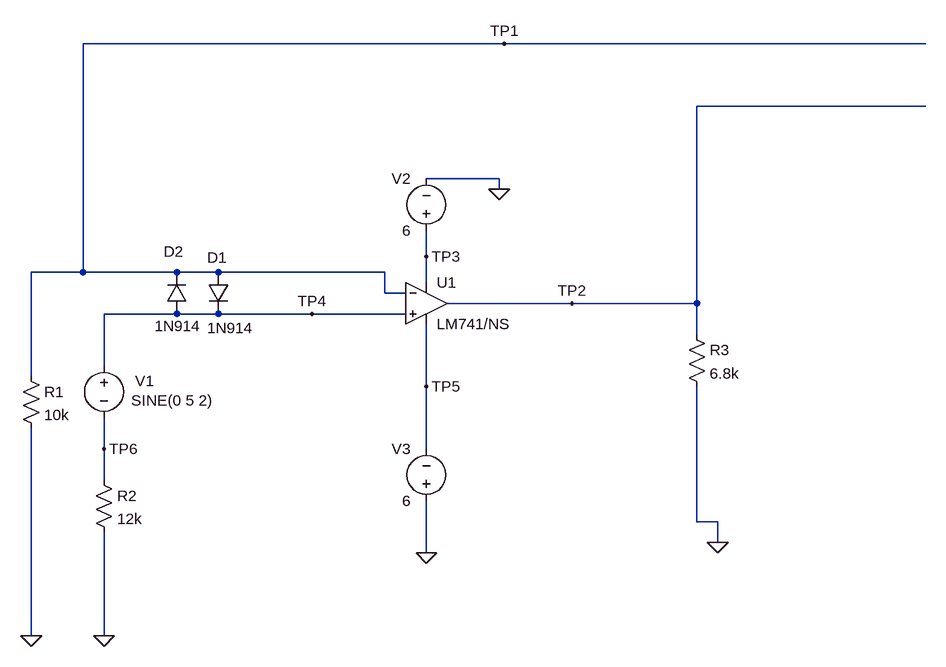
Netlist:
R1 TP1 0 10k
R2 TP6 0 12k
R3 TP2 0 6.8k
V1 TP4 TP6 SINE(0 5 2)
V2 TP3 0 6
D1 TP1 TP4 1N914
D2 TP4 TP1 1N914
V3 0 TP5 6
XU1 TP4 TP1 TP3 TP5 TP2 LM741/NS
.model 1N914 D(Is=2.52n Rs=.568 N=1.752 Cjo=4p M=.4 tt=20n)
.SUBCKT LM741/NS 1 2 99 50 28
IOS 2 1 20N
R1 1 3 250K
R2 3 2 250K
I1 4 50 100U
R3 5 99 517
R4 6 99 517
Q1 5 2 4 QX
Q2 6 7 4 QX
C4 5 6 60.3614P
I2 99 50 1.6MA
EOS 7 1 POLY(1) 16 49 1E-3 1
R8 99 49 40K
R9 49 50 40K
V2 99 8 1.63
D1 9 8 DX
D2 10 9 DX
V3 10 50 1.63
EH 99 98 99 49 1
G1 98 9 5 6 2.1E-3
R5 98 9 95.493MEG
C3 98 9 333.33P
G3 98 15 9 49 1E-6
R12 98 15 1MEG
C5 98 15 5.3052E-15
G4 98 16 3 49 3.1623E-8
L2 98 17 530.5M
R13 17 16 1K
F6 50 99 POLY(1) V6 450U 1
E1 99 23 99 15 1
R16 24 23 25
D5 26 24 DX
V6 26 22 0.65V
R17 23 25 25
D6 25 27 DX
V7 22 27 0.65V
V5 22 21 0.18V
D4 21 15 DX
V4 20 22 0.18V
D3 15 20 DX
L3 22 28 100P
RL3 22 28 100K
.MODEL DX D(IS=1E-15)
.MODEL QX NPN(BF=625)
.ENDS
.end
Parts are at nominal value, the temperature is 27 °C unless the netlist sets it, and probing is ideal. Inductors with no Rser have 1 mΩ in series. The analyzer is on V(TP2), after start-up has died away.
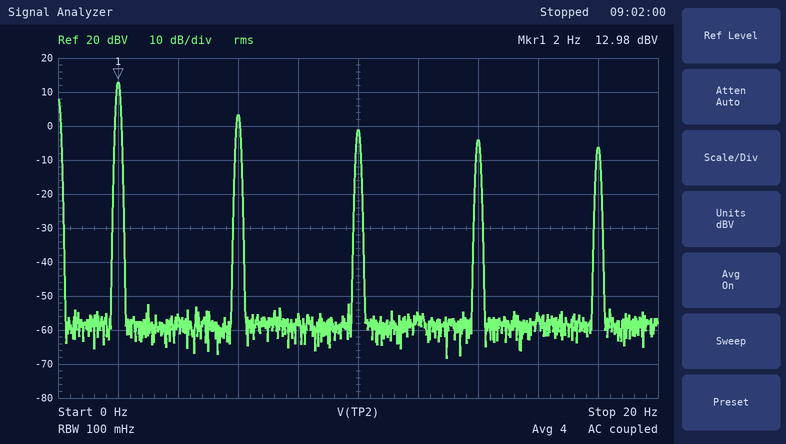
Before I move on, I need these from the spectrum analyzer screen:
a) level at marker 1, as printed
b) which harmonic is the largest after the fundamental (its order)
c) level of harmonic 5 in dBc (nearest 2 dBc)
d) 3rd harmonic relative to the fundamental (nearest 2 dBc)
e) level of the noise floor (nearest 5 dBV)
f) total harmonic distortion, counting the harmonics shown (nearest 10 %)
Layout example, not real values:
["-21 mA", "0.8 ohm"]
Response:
["12.98 dBV", "3", "-14 dBc", "-10 dBc", "-60 dBV", "40 %"]
